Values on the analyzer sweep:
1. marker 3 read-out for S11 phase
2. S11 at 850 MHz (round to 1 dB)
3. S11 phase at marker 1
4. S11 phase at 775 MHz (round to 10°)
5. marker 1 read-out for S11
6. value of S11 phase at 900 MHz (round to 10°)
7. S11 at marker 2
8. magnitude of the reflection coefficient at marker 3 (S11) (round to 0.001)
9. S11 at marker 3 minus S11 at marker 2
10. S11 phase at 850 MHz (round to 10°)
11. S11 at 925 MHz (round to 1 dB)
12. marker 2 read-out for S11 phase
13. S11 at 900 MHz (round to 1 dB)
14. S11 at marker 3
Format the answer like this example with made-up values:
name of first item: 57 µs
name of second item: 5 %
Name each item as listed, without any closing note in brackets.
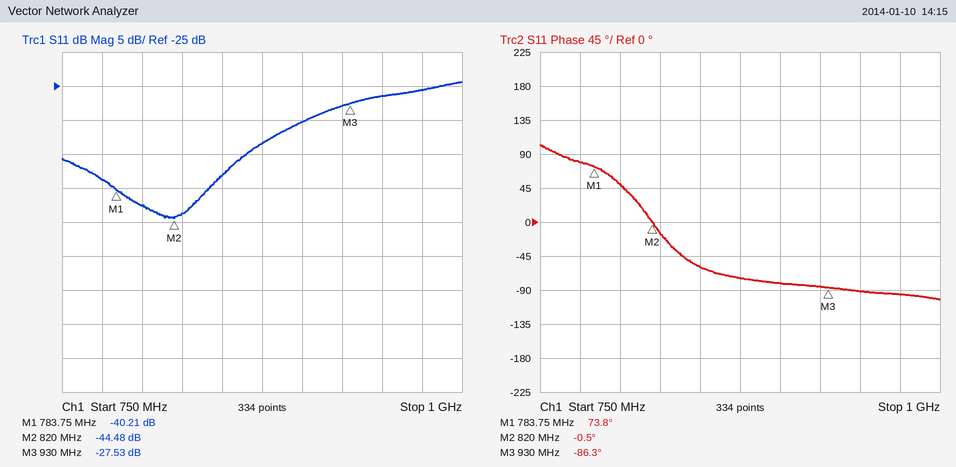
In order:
marker 3 read-out for S11 phase: -86.3°
S11 at 850 MHz: -38 dB
S11 phase at marker 1: 73.8°
S11 phase at 775 MHz: 80°
marker 1 read-out for S11: -40.21 dB
value of S11 phase at 900 MHz: -80°
S11 at marker 2: -44.48 dB
magnitude of the reflection coefficient at marker 3 (S11): 0.042
S11 at marker 3 minus S11 at marker 2: 16.95 dB
S11 phase at 850 MHz: -60°
S11 at 925 MHz: -28 dB
marker 2 read-out for S11 phase: -0.5°
S11 at 900 MHz: -30 dB
S11 at marker 3: -27.53 dB
